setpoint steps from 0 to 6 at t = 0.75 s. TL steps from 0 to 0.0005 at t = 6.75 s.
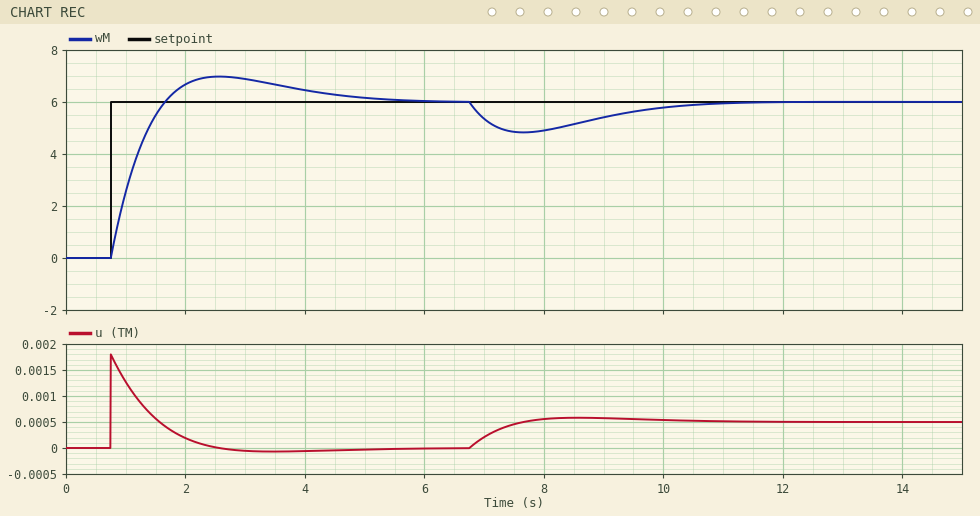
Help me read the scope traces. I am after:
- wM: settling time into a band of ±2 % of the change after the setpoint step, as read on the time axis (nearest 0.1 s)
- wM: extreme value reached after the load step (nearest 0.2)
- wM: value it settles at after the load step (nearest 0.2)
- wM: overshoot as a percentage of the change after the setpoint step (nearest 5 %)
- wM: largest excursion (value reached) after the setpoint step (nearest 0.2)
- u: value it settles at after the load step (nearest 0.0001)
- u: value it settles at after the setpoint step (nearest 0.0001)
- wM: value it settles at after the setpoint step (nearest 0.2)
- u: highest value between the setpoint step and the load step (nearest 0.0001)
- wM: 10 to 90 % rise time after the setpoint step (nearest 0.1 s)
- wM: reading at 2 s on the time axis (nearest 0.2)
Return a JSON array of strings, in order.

["5.2 s", "4.8", "6.0", "15 %", "7.0", "0.0005", "0.0000", "6.0", "0.0018", "0.7 s", "6.6"]
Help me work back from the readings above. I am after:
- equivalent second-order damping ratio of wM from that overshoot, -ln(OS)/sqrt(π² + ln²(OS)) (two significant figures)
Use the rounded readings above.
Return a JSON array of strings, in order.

["0.52"]
